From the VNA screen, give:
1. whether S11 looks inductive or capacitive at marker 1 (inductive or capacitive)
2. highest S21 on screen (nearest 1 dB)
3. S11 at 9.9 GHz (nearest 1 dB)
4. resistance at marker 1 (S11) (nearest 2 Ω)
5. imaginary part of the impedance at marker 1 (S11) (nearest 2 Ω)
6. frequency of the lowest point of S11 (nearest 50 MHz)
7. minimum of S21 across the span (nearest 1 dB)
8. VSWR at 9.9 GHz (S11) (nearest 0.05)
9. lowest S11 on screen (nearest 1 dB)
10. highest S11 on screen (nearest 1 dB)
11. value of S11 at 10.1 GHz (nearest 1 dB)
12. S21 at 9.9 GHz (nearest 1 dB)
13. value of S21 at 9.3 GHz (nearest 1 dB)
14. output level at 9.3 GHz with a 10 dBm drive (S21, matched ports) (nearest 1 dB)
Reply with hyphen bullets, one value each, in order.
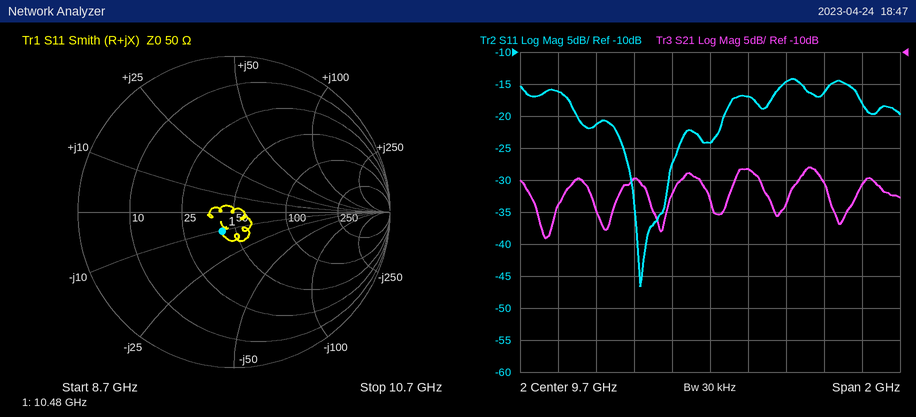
- capacitive
- -28 dB
- -17 dB
- 42 Ω
- -10 Ω
- 9.35 GHz
- -39 dB
- 1.35
- -47 dB
- -14 dB
- -15 dB
- -28 dB
- -30 dB
- -20 dBm
